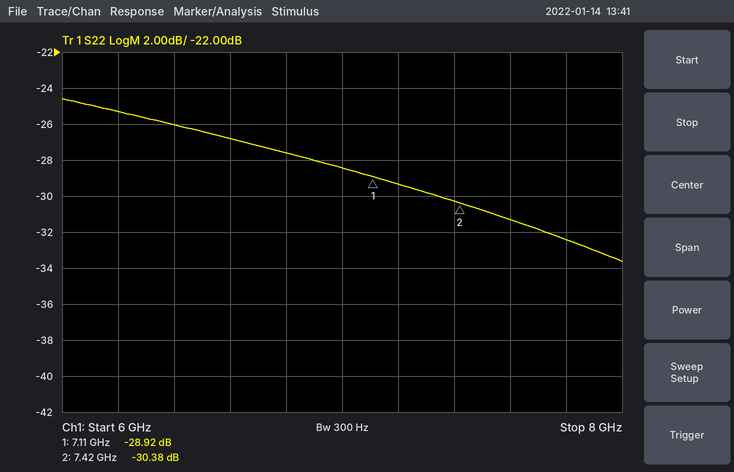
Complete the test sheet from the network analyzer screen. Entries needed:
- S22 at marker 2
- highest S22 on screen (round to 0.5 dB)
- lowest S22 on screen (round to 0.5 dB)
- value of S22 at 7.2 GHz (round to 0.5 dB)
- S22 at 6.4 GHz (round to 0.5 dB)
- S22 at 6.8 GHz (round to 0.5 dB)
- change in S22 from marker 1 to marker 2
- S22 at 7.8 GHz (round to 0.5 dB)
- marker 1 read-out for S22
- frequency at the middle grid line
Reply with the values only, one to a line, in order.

-30.38 dB
-24.5 dB
-33.5 dB
-29.5 dB
-26.0 dB
-27.5 dB
-1.46 dB
-32.5 dB
-28.92 dB
7 GHz
